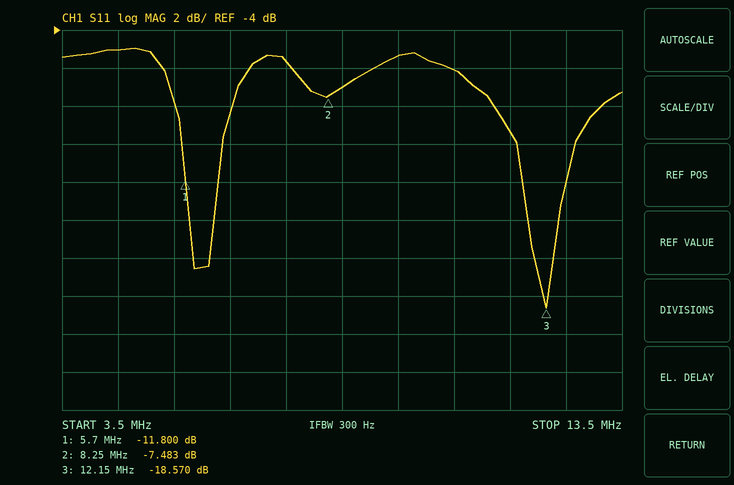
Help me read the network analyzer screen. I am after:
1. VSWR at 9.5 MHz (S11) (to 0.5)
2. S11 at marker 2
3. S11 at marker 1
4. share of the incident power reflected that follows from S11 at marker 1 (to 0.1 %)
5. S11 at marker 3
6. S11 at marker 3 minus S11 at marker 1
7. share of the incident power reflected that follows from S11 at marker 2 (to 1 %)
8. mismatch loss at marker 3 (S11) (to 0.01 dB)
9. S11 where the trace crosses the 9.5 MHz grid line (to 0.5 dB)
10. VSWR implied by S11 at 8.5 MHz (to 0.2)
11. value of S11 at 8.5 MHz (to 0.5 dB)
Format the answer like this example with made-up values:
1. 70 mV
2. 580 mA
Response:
1. 3.5
2. -7.483 dB
3. -11.800 dB
4. 6.6 %
5. -18.570 dB
6. -6.770 dB
7. 18 %
8. 0.06 dB
9. -5.5 dB
10. 2.6
11. -7.0 dB
